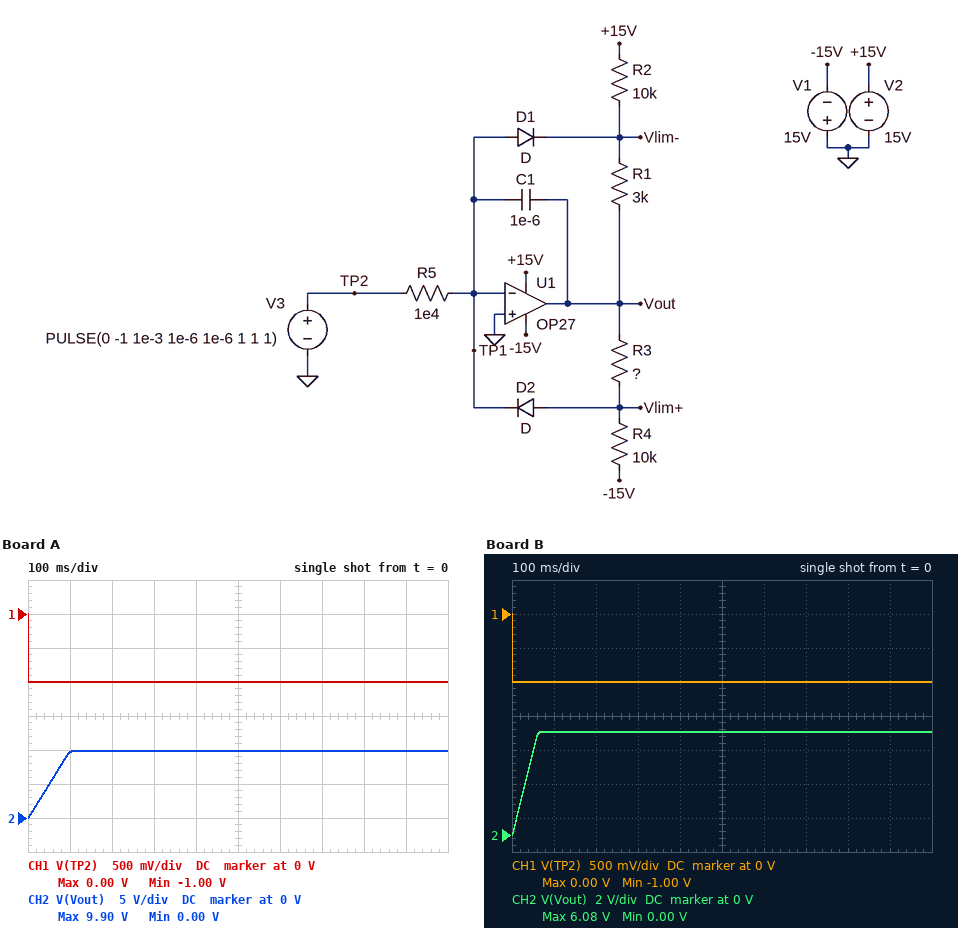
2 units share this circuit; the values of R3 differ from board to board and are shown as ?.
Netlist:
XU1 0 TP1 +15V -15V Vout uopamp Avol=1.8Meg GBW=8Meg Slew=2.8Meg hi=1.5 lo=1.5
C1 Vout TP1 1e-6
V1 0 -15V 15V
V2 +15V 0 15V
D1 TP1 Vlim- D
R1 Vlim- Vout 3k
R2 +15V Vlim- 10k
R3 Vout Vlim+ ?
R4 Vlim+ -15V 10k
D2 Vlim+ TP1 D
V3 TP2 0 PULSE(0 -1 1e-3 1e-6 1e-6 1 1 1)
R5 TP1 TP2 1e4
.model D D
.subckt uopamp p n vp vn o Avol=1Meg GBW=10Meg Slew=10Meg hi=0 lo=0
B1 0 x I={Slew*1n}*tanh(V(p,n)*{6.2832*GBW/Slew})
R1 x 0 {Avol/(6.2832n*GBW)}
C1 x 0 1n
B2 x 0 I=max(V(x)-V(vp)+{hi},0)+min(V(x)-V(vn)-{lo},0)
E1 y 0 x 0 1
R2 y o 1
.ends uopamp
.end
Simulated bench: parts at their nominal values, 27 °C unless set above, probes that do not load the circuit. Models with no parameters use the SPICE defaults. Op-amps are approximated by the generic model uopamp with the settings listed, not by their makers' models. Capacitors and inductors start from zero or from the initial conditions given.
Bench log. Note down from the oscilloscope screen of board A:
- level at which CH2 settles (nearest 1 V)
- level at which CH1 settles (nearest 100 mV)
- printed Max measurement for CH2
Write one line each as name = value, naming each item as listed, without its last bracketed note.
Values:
level at which CH2 settles = 10 V
level at which CH1 settles = -1.0 V
printed Max measurement for CH2 = 9.90 V
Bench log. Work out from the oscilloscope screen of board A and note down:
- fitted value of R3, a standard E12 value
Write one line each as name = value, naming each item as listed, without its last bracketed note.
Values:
fitted value of R3, a standard E12 value = 5.6 kΩ
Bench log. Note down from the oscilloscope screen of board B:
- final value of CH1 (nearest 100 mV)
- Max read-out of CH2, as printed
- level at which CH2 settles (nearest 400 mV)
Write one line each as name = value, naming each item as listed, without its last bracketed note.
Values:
final value of CH1 = -1.0 V
Max read-out of CH2, as printed = 6.08 V
level at which CH2 settles = 6.0 V
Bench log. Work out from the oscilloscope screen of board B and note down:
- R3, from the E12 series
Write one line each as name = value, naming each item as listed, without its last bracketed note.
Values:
R3, from the E12 series = 3.3 kΩ
